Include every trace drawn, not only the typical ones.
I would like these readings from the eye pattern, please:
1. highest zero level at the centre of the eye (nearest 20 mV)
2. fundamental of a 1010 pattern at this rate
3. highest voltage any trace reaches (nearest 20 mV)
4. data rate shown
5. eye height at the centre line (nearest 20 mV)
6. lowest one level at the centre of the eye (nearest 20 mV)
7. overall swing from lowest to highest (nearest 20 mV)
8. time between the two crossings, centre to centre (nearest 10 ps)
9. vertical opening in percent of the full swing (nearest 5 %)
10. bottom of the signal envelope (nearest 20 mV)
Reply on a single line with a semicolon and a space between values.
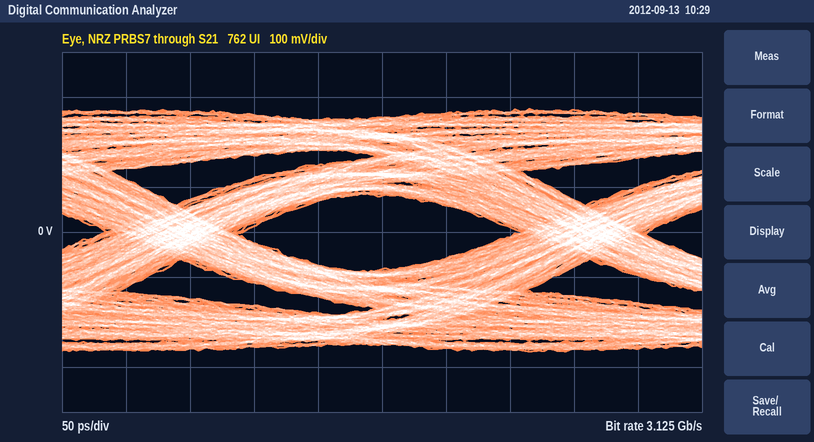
-80 mV; 1.5625 GHz; 280 mV; 3.125 Gb/s; 160 mV; 80 mV; 540 mV; 320 ps; 30 %; -260 mV
